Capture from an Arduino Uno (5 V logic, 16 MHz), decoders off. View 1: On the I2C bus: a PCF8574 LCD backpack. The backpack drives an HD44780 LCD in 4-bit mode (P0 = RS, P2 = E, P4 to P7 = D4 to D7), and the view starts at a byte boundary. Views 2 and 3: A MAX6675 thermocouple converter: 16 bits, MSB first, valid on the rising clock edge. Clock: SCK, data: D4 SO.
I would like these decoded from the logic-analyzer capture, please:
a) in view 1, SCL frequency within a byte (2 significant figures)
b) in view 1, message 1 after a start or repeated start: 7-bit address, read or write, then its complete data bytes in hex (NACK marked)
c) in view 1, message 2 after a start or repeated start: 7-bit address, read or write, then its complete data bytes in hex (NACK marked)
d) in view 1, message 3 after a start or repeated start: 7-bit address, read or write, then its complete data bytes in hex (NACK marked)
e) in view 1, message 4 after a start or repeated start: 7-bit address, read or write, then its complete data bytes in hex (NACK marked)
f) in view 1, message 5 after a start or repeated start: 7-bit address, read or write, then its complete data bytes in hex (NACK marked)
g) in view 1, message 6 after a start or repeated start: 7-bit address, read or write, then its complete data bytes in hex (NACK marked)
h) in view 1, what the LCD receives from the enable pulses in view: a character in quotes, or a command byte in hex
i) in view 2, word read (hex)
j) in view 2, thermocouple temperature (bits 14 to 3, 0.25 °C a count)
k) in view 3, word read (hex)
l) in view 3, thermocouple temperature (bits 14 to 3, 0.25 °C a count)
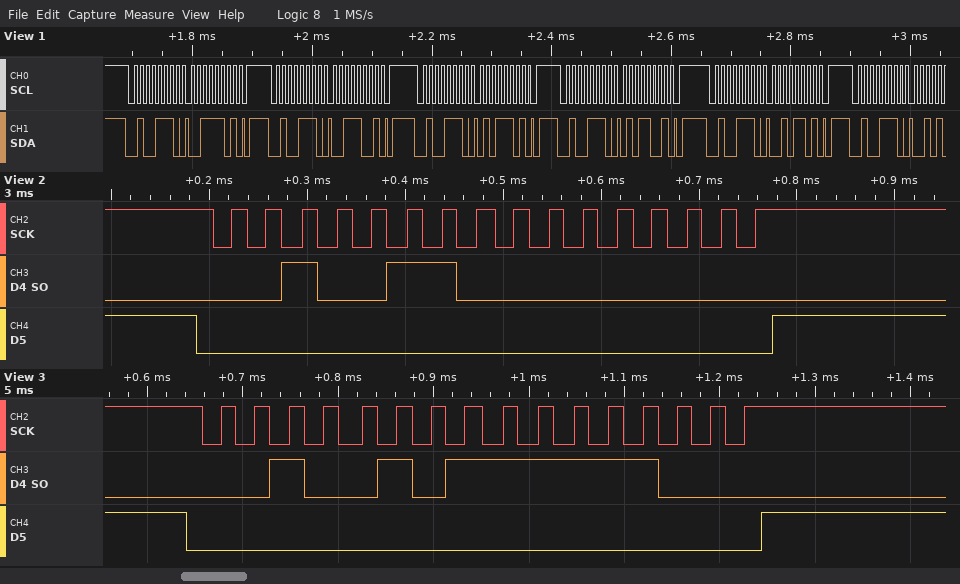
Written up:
100 kHz
0x27 write: 3D
0x27 write: 39
0x27 write: 5D
0x27 write: 59
0x27 write: 2D
0x27 write
'5'
0x2600
304.00 °C
0x25F8
303.75 °C
